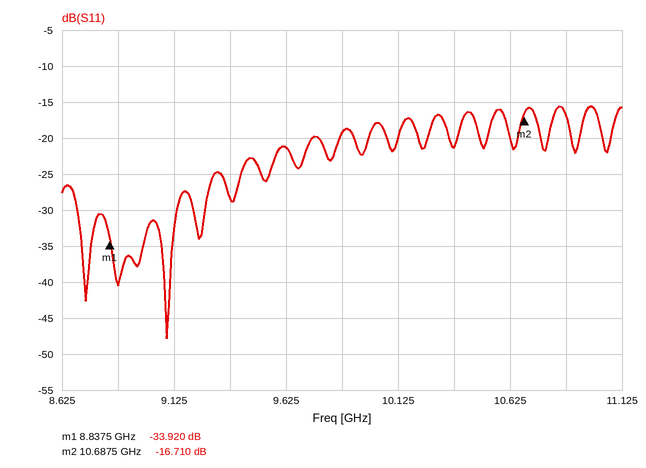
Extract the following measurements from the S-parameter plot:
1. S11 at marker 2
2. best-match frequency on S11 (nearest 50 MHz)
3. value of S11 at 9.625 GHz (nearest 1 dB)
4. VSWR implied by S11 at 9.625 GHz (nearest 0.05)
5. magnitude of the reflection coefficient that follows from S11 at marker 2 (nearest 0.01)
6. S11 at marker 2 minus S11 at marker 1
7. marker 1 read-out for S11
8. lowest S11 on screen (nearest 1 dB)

-16.710 dB
9.10 GHz
-21 dB
1.20
0.15
17.210 dB
-33.920 dB
-48 dB
